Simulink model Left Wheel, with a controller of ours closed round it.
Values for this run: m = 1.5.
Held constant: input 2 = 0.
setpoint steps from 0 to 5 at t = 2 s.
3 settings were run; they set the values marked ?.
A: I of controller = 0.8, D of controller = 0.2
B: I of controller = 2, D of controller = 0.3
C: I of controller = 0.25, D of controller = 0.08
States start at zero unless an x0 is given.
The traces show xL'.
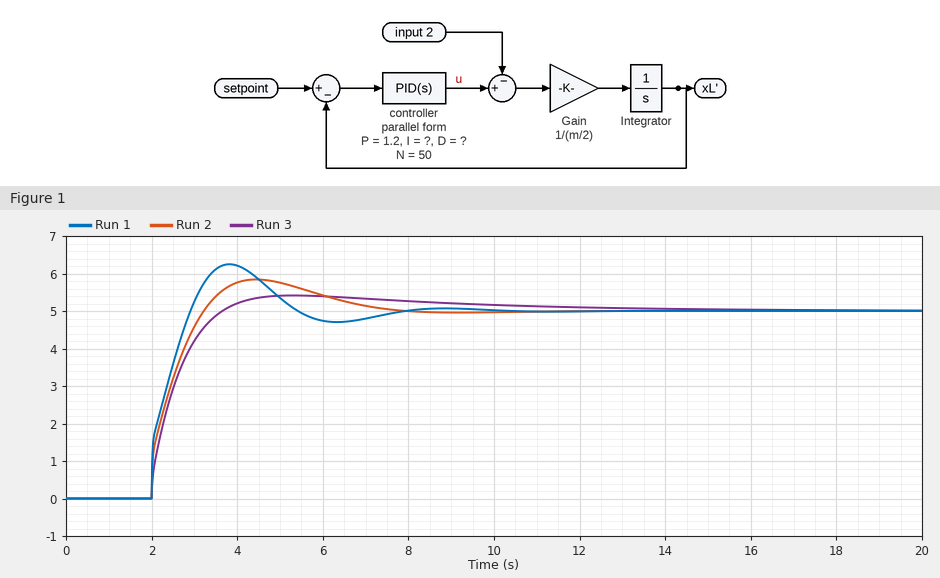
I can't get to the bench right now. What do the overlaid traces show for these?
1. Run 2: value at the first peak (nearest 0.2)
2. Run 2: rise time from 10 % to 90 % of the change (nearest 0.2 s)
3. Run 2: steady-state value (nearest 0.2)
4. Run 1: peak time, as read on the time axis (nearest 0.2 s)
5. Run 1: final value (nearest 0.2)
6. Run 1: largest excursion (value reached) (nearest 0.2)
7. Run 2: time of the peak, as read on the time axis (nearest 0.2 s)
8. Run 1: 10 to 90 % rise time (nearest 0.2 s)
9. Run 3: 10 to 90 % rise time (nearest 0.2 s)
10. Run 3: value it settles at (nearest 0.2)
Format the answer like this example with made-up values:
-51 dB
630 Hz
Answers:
5.8
1.0 s
5.0
3.8 s
5.0
6.2
4.4 s
0.8 s
1.2 s
5.0
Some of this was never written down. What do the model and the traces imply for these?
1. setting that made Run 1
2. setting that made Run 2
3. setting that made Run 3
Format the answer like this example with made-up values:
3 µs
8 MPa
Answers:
B
A
C
